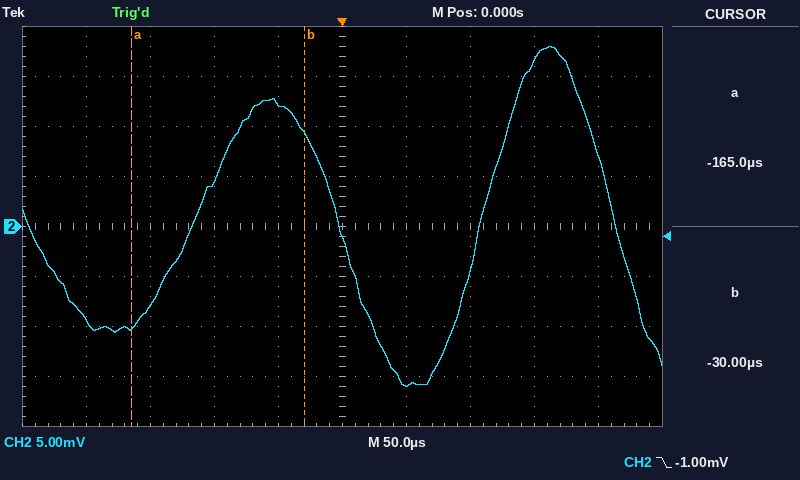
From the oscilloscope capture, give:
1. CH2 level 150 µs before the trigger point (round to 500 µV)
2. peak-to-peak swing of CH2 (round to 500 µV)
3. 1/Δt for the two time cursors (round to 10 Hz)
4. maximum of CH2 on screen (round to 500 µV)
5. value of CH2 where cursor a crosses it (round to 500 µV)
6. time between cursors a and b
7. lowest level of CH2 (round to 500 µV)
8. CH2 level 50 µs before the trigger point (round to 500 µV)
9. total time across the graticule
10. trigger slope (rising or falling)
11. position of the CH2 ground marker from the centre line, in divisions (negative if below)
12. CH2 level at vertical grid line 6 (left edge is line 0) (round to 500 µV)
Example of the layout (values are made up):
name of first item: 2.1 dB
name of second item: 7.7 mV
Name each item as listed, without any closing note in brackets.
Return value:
CH2 level 150 µs before the trigger point: -8.0 mV
peak-to-peak swing of CH2: 34.0 mV
1/Δt for the two time cursors: 7.41 kHz
maximum of CH2 on screen: 18.0 mV
value of CH2 where cursor a crosses it: -10.0 mV
time between cursors a and b: 135 µs
lowest level of CH2: -16.0 mV
CH2 level 50 µs before the trigger point: 12.5 mV
total time across the graticule: 500 µs
trigger slope: falling
position of the CH2 ground marker from the centre line, in divisions: 0.0 div
CH2 level at vertical grid line 6 (left edge is line 0): -16.0 mV
